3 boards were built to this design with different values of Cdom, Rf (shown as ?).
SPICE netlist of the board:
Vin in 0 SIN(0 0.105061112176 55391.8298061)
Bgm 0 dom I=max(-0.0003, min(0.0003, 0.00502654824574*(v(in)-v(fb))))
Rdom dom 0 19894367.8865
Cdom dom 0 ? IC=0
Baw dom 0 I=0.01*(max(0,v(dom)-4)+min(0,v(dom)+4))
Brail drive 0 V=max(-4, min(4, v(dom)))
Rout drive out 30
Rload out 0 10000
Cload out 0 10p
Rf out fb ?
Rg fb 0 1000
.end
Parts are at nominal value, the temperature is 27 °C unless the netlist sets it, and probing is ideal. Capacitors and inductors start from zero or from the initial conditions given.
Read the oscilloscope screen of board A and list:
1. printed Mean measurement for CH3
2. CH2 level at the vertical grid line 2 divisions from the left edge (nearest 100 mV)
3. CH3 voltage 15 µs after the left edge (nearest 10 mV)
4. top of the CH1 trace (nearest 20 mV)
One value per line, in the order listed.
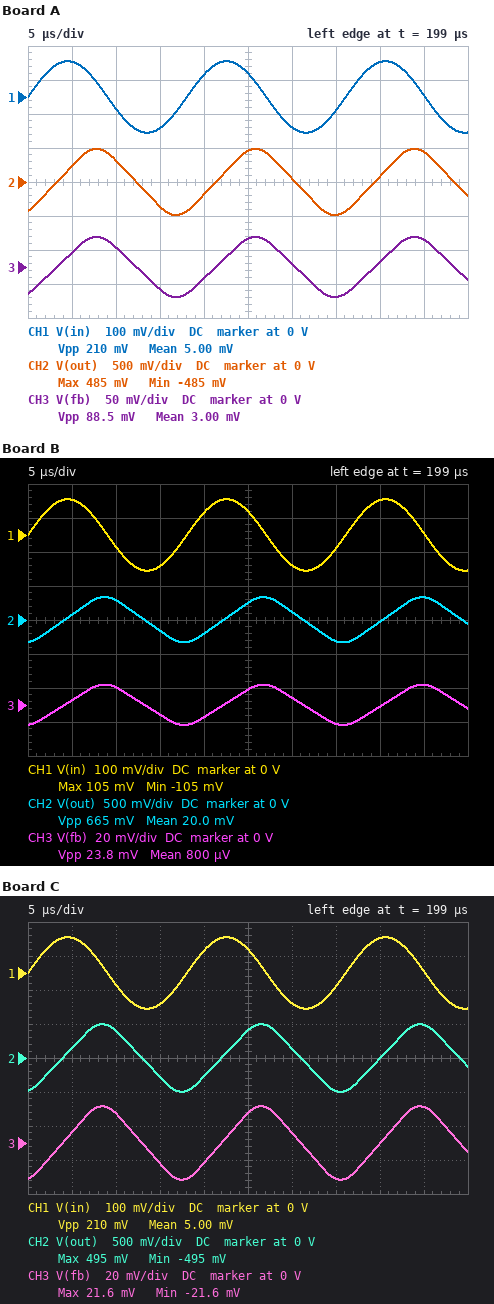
3.00 mV
300 mV
-30 mV
100 mV
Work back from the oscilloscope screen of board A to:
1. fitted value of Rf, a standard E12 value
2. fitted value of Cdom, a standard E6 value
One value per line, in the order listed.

10 kΩ
2.2 nF
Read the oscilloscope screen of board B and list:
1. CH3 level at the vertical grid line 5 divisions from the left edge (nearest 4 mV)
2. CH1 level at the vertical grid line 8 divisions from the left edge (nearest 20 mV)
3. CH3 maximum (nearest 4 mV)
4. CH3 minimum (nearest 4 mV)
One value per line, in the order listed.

8 mV
100 mV
12 mV
-12 mV
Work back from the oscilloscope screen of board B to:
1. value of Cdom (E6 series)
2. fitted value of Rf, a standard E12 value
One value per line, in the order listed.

3.3 nF
27 kΩ
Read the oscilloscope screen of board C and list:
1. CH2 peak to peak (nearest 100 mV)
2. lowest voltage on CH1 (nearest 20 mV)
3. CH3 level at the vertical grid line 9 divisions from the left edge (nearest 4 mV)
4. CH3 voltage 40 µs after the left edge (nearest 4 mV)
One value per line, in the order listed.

1.0 V
-100 mV
20 mV
0 V
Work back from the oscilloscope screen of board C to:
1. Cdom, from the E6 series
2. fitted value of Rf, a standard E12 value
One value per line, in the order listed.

2.2 nF
22 kΩ
